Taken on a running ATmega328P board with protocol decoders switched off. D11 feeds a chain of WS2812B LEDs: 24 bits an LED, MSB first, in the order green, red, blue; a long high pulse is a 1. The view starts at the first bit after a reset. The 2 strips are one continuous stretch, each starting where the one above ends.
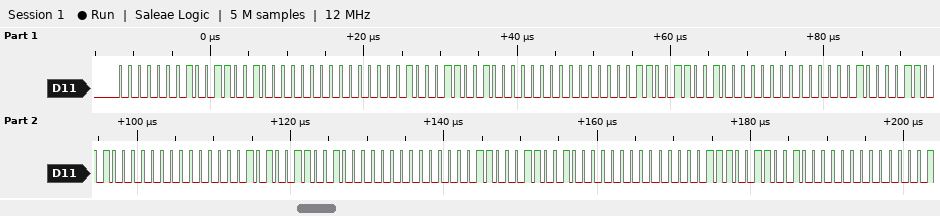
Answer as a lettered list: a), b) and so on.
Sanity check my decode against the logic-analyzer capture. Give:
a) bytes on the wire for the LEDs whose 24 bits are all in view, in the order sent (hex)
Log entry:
a) 01 32 00 02 32 00 03 32 00 04 32 00 05 32 00 06 32 00 07 32 00
